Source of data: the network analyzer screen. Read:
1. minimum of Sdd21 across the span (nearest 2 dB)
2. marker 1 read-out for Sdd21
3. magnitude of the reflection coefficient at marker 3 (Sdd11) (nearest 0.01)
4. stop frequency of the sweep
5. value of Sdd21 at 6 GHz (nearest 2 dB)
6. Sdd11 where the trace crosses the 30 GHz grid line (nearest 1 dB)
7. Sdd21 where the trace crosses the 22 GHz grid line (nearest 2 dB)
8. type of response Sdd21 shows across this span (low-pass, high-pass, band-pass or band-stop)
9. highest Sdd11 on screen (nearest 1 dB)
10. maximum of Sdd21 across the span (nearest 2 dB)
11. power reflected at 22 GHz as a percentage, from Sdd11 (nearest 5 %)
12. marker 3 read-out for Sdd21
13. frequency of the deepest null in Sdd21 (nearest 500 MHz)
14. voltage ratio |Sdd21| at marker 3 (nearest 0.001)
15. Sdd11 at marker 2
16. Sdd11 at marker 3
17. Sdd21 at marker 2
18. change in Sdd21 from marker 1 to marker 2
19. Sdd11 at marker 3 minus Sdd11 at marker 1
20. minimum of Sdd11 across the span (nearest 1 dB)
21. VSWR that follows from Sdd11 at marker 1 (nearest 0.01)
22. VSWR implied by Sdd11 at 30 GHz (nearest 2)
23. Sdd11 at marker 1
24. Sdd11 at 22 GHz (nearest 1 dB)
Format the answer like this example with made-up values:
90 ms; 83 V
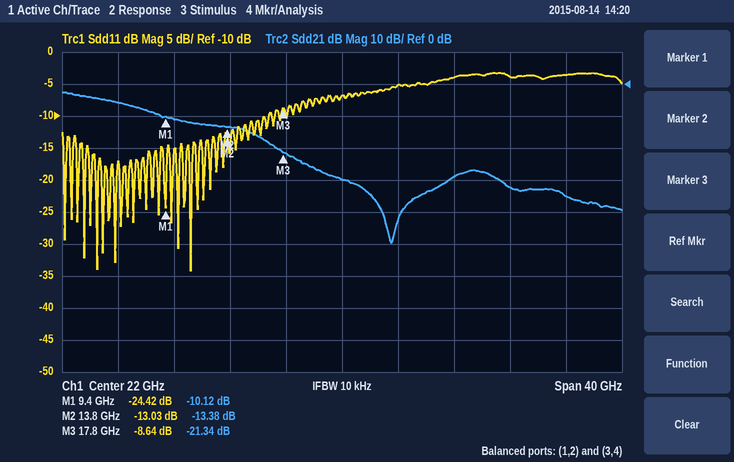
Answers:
-50 dB; -10.12 dB; 0.37; 42 GHz; -6 dB; -4 dB; -30 dB; low-pass; -3 dB; -2 dB; 20 %; -21.34 dB; 25.5 GHz; 0.086; -13.03 dB; -8.64 dB; -13.38 dB; -3.26 dB; 15.78 dB; -34 dB; 1.13; 4; -24.42 dB; -7 dB
